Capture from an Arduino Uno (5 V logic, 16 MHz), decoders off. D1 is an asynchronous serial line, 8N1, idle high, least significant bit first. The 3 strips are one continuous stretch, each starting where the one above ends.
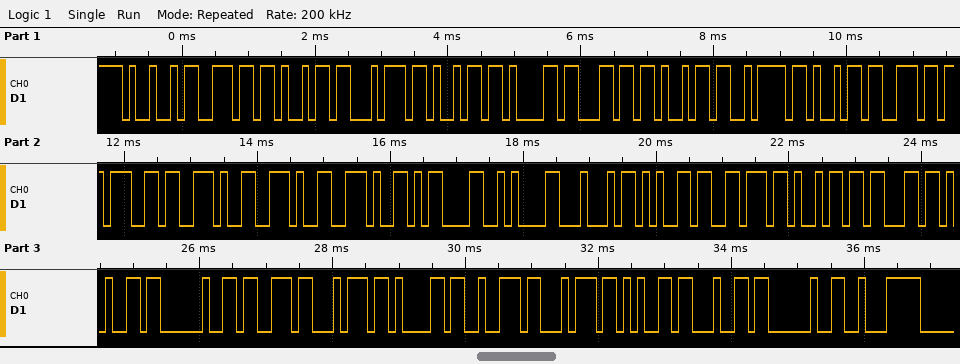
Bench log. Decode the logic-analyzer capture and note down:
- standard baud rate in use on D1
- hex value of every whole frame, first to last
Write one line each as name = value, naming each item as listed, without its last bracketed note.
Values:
standard baud rate in use on D1 = 9600 baud
hex value of every whole frame, first to last = 49 6E 69 74 69 61 6C 69 7A 69 6E 67 2E 2E 2E 0D 0A 44 65 76 69 63 65 20 73 74 61 72 74 65 64 20 E2
